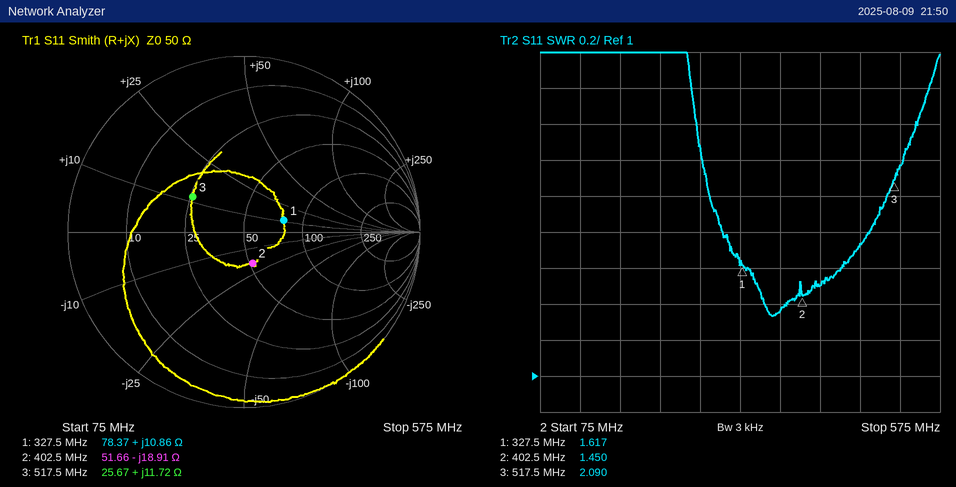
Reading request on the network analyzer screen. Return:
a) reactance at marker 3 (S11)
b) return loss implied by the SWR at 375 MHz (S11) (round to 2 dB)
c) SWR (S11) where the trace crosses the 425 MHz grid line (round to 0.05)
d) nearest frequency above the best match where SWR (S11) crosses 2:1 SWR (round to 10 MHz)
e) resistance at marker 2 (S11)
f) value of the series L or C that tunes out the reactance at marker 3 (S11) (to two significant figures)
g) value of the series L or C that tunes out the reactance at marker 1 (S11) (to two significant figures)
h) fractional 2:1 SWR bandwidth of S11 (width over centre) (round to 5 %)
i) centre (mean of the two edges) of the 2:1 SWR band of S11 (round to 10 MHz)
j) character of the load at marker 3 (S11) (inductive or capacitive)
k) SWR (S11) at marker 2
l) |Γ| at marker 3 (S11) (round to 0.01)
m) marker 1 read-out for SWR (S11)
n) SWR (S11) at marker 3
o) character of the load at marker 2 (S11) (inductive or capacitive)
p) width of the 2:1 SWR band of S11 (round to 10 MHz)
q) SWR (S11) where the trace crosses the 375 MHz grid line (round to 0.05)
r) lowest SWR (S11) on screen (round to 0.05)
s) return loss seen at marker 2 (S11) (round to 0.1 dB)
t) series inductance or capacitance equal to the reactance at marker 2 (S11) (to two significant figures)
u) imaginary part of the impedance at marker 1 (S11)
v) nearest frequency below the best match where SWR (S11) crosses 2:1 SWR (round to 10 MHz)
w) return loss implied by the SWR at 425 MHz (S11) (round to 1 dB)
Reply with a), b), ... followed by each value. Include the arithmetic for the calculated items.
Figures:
a) +11.72 Ω
b) −20 log10((1.35 − 1)/(1.35 + 1)) ≈ 16 dB
c) 1.50
d) 510 MHz
e) 51.66 Ω
f) C = 1/(2π × 517.5 MHz × 11.72 Ω) ≈ 26 pF
g) C = 1/(2π × 327.5 MHz × 10.86 Ω) ≈ 45 pF
h) 220 MHz / 400 MHz ≈ 55 %
i) 400 MHz
j) inductive
k) 1.450
l) 0.35
m) 1.617
n) 2.090
o) capacitive
p) 510 MHz − 290 MHz = 220 MHz
q) 1.35
r) 1.35
s) 14.7 dB
t) C = 1/(2π × 402.5 MHz × 18.91 Ω) ≈ 21 pF
u) +10.86 Ω
v) 290 MHz
w) −20 log10((1.5 − 1)/(1.5 + 1)) ≈ 14 dB
